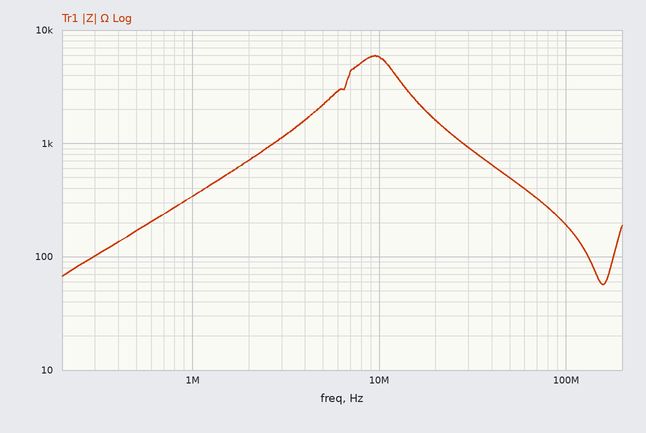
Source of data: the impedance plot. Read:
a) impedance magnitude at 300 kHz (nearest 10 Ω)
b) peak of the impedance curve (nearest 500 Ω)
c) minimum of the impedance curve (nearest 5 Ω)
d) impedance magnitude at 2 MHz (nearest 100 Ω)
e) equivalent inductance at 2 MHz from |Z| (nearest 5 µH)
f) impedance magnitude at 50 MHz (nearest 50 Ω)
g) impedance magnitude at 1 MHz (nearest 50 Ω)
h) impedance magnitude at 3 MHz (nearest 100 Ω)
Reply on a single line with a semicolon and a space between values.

100 Ω; 6.0 kΩ; 55 Ω; 700 Ω; 55 µH; 500 Ω; 350 Ω; 1.1 kΩ
